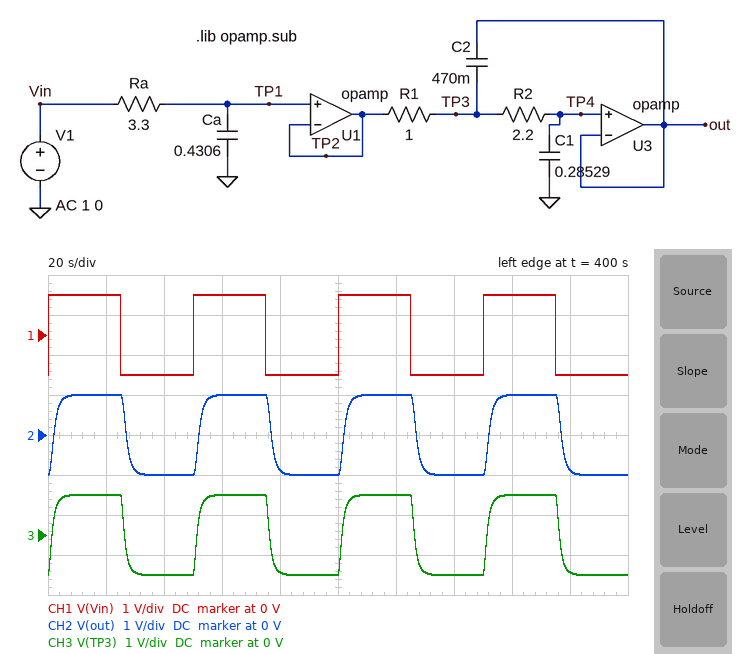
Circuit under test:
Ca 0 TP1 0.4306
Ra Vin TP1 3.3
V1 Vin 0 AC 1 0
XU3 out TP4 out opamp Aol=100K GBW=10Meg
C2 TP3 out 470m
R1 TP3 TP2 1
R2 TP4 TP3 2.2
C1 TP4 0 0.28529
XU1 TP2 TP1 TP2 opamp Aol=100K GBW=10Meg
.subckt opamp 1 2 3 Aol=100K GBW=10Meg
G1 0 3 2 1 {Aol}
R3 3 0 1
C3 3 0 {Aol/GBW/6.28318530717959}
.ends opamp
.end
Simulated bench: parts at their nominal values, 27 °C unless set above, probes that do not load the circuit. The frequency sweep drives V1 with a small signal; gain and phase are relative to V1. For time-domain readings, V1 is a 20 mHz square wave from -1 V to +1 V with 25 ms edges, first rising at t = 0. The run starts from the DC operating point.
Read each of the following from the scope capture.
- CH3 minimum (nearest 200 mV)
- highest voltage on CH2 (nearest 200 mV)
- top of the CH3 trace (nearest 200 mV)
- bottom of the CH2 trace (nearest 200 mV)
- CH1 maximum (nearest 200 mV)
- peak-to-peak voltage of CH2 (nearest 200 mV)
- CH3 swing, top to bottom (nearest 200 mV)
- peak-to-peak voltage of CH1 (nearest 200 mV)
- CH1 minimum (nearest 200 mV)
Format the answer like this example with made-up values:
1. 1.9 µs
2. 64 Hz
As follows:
1. -1.0 V
2. 1.0 V
3. 1.0 V
4. -1.0 V
5. 1.0 V
6. 2.0 V
7. 2.0 V
8. 2.0 V
9. -1.0 V
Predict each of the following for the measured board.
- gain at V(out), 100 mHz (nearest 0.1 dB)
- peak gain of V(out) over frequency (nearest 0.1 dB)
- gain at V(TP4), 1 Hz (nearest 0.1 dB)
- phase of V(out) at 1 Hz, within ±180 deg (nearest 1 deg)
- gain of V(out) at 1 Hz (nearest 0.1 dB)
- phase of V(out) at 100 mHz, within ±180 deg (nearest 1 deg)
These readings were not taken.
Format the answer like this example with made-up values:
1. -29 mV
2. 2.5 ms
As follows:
1. -3.0 dB
2. 0 dB
3. -40.7 dB
4. 125 deg
5. -40.7 dB
6. -75 deg
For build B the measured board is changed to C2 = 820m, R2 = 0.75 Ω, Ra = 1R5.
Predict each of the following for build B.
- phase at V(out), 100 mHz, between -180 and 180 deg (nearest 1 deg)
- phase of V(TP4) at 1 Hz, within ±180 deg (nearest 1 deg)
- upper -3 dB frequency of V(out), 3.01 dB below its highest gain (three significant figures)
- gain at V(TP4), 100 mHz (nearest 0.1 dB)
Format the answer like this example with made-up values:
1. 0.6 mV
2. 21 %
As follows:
1. -41 deg
2. 132 deg
3. 260 mHz
4. -0.5 dB
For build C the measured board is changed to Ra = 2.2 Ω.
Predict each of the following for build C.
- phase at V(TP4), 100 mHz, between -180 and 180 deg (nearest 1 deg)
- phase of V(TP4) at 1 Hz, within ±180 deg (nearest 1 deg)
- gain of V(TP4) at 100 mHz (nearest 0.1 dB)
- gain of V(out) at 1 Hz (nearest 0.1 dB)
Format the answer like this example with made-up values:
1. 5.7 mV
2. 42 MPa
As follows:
1. -64 deg
2. 128 deg
3. -1.8 dB
4. -37.3 dB
